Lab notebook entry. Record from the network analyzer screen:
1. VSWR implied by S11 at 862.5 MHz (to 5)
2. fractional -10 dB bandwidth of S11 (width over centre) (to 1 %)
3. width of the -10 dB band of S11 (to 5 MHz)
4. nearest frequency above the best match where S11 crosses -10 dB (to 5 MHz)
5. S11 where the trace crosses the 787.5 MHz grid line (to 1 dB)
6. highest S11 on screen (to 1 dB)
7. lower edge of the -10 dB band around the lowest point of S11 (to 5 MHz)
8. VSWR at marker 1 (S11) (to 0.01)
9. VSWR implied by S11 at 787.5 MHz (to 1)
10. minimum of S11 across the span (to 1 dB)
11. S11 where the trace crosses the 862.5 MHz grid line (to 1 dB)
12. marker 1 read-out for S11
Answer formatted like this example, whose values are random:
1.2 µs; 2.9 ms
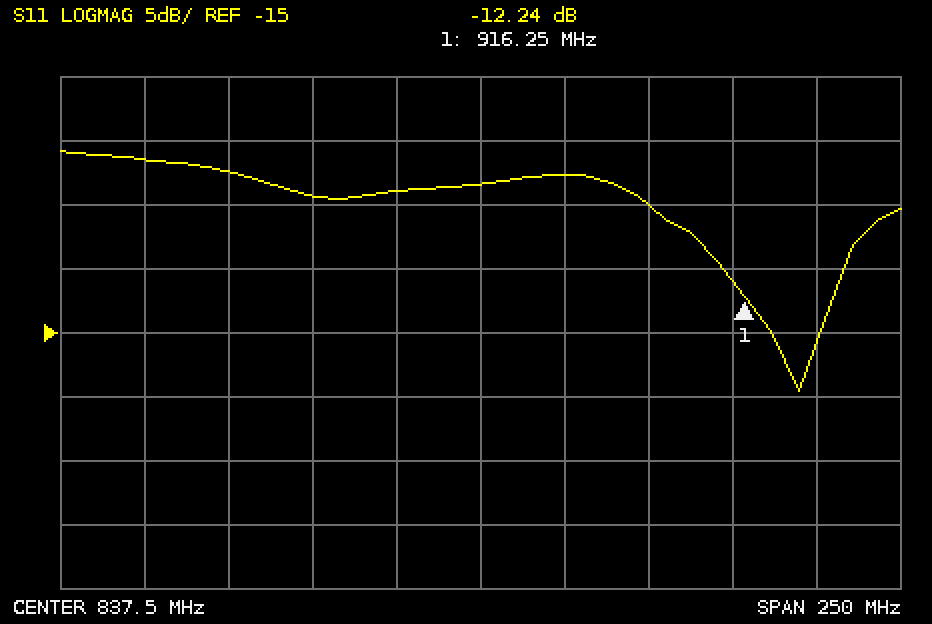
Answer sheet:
5; 4 %; 35 MHz; 945 MHz; -4 dB; -1 dB; 910 MHz; 1.65; 4; -20 dB; -3 dB; -12.24 dB
